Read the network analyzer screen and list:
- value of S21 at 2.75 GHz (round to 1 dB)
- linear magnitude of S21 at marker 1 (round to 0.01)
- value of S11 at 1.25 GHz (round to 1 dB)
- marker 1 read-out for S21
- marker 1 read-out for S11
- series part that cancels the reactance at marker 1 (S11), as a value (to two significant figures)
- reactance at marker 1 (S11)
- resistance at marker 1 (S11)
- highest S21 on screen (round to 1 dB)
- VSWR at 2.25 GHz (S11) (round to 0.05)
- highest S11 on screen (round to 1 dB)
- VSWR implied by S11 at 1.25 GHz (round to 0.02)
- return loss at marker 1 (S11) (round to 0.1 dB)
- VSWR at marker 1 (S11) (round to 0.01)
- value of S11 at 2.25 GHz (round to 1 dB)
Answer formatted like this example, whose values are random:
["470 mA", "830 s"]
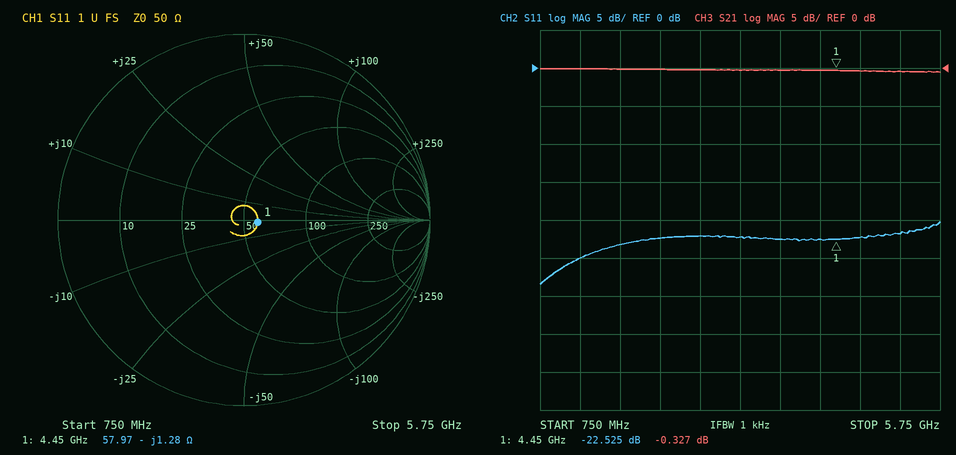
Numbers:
["0 dB", "0.96", "-25 dB", "-0.327 dB", "-22.525 dB", "46 pH", "-1.28 Ω", "57.97 Ω", "0 dB", "1.15", "-20 dB", "1.12", "22.5 dB", "1.16", "-22 dB"]
